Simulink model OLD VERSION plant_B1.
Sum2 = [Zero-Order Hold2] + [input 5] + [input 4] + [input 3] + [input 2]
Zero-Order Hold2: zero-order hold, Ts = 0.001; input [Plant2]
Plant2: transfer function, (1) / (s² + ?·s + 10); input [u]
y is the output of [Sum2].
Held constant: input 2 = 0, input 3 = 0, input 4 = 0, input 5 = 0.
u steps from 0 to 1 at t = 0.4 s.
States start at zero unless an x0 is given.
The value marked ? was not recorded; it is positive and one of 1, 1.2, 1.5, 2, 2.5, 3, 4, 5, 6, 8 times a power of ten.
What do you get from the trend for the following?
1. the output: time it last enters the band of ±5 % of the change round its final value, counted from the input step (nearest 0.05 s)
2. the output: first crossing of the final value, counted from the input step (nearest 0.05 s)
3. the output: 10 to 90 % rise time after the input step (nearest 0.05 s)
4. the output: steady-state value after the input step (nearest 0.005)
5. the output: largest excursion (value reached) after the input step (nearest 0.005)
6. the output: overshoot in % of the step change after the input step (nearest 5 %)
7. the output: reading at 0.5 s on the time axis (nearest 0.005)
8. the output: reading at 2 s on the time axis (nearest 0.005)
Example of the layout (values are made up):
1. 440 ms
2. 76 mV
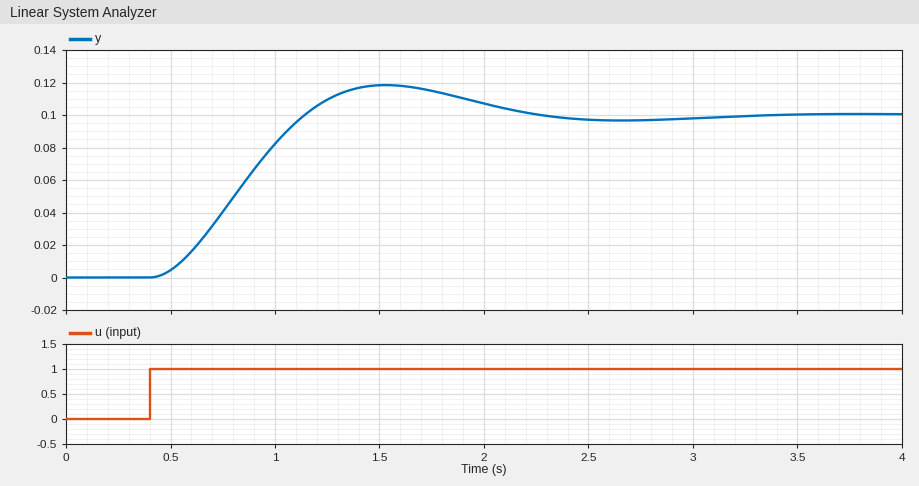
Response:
1. 1.65 s
2. 0.75 s
3. 0.50 s
4. 0.100
5. 0.120
6. 20 %
7. 0.005
8. 0.105
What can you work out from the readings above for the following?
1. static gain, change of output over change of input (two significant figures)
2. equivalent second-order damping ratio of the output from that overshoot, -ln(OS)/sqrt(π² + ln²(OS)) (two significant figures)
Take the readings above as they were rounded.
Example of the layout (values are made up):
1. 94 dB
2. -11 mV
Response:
1. 0.10
2. 0.46
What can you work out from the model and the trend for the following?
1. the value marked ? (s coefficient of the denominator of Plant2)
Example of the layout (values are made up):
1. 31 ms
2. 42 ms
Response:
1. 3
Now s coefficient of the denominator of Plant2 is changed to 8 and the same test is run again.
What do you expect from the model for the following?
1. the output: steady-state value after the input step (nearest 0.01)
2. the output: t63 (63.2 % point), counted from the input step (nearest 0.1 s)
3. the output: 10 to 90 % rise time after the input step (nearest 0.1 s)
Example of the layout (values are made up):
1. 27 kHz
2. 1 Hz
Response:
1. 0.10
2. 0.8 s
3. 1.5 s
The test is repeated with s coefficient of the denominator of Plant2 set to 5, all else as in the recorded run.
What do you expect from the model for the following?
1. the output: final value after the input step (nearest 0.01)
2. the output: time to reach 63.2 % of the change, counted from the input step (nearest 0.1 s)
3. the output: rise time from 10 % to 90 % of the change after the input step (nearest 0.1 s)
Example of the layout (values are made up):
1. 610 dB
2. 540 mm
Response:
1. 0.10
2. 0.6 s
3. 0.8 s
